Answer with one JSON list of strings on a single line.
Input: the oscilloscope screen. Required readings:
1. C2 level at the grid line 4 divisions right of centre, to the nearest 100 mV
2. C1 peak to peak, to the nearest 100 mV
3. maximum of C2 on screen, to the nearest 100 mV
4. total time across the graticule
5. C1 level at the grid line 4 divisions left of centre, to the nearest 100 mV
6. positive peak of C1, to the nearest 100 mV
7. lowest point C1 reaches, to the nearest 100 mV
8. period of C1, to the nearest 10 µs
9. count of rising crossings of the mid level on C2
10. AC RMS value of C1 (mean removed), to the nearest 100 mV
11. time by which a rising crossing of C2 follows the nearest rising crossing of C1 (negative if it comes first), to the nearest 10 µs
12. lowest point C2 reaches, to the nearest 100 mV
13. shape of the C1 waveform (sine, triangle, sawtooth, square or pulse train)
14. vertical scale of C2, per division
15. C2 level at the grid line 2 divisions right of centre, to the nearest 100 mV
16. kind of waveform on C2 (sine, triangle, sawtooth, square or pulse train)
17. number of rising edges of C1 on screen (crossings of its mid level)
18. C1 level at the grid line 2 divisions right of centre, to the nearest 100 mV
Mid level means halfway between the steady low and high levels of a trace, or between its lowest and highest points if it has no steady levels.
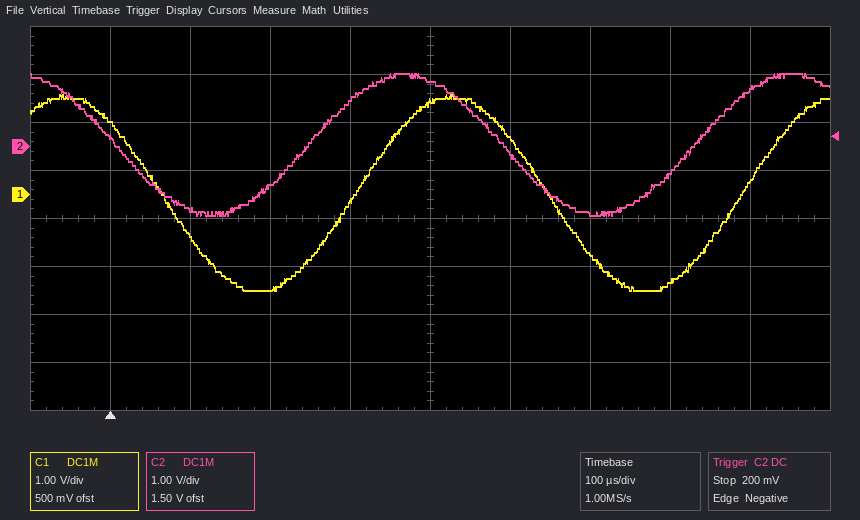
["1.2 V", "4.1 V", "1.5 V", "1 ms", "1.5 V", "2.1 V", "-2.0 V", "480 µs", "2", "1.4 V", "-60 µs", "-1.4 V", "sine", "1 V", "-1.4 V", "sine", "2", "-1.3 V"]
